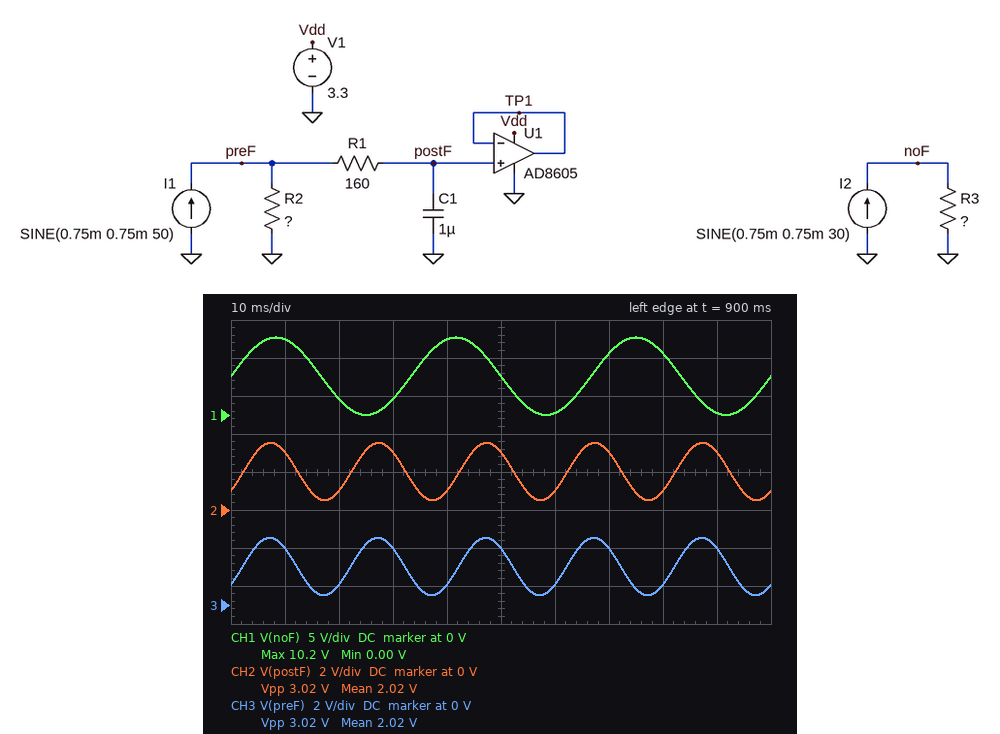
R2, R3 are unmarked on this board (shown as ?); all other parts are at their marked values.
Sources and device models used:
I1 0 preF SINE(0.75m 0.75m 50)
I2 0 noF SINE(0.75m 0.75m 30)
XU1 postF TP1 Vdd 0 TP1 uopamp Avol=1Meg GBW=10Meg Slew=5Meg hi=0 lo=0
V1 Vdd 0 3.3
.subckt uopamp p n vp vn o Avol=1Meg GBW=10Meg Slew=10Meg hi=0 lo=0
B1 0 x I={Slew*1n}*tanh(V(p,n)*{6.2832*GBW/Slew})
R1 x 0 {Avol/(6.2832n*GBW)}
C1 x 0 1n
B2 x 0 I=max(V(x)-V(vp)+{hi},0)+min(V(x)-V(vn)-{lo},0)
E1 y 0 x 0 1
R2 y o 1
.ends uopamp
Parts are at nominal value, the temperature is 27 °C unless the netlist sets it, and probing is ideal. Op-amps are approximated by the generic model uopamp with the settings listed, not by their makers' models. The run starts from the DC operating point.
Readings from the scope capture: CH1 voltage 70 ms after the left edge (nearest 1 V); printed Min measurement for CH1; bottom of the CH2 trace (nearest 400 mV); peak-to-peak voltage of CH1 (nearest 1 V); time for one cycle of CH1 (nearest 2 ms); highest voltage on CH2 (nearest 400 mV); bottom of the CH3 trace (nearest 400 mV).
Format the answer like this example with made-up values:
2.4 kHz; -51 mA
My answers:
8 V; 0.00 V; 400 mV; 10 V; 34 ms; 3.6 V; 400 mV
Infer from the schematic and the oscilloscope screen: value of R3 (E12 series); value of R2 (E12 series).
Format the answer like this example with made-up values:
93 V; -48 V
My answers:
6.8 kΩ; 2.7 kΩ
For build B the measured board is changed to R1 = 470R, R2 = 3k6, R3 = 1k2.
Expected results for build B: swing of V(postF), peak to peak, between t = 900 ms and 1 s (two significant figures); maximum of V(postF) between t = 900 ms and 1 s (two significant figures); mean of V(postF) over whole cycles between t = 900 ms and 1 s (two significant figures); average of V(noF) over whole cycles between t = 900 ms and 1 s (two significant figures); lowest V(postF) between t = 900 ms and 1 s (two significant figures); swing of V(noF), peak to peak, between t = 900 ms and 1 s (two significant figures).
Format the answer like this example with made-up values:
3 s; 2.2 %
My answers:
3.3 V; 4.4 V; 2.7 V; 900 mV; 1.0 V; 1.8 V
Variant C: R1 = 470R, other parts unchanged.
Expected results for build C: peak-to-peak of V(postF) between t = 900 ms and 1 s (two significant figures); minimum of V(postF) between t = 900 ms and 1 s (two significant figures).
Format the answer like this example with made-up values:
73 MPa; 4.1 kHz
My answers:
2.9 V; 590 mV
